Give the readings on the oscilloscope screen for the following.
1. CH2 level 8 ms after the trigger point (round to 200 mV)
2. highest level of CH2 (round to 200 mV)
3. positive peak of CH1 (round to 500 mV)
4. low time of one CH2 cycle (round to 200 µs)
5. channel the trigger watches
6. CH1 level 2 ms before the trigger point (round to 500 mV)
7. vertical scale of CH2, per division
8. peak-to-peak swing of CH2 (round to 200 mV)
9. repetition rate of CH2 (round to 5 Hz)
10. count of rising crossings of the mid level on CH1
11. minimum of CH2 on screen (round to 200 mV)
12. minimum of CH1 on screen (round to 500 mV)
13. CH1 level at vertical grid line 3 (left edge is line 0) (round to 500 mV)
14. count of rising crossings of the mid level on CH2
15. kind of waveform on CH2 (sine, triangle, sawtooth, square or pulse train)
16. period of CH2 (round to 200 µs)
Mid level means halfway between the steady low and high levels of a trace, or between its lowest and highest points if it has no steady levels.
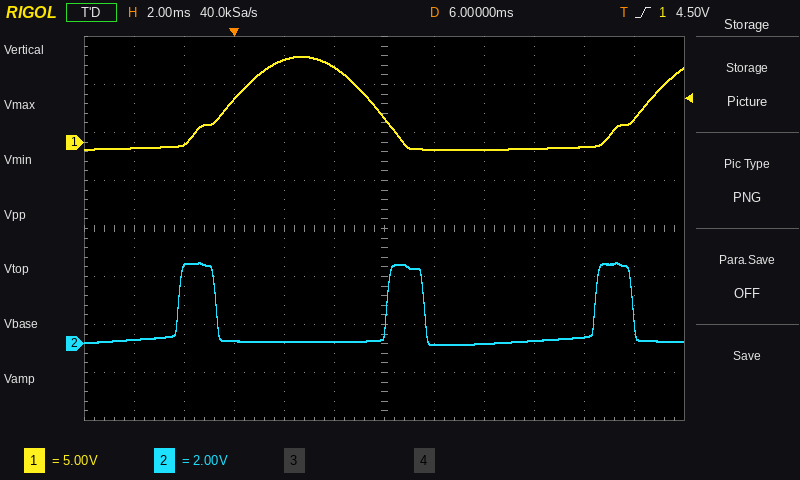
0.0 V
3.4 V
9.0 V
6.8 ms
CH1
0.0 V
2 V
3.4 V
120 Hz
2
0.0 V
-1.0 V
4.5 V
3
pulse train
8.4 ms
